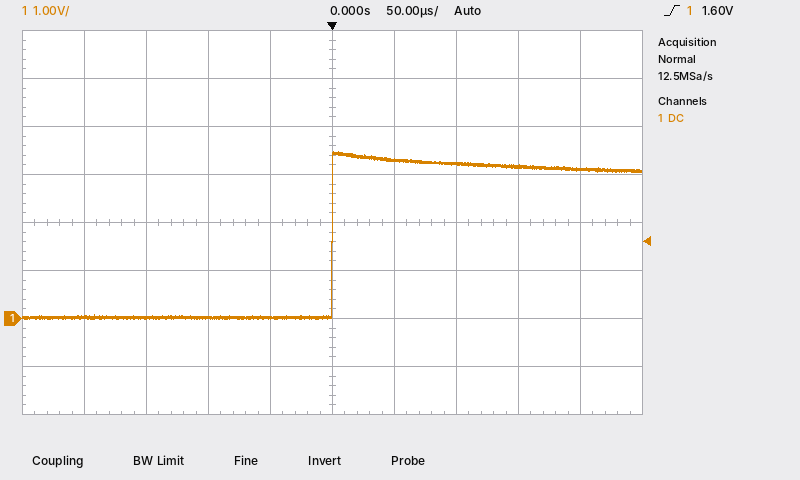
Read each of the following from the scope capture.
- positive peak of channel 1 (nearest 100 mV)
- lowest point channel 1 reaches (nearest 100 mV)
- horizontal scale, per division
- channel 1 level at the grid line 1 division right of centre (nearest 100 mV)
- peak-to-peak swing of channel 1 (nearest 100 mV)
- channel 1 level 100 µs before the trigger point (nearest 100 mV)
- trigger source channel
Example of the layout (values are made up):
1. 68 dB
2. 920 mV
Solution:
1. 3.5 V
2. 0.0 V
3. 50 µs
4. 3.3 V
5. 3.5 V
6. 0.0 V
7. channel 1
